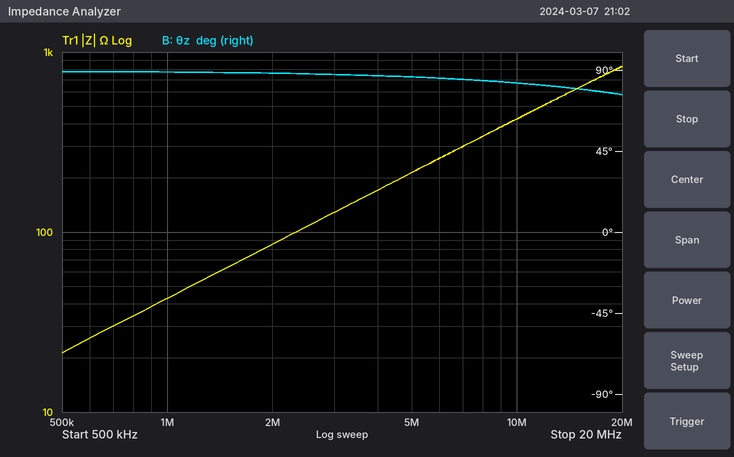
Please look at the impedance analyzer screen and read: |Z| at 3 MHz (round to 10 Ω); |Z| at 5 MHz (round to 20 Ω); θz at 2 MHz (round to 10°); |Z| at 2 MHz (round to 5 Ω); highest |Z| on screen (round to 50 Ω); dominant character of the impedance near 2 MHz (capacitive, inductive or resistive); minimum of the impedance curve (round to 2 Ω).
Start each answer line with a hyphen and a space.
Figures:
- 130 Ω
- 220 Ω
- 90°
- 85 Ω
- 850 Ω
- inductive
- 22 Ω
